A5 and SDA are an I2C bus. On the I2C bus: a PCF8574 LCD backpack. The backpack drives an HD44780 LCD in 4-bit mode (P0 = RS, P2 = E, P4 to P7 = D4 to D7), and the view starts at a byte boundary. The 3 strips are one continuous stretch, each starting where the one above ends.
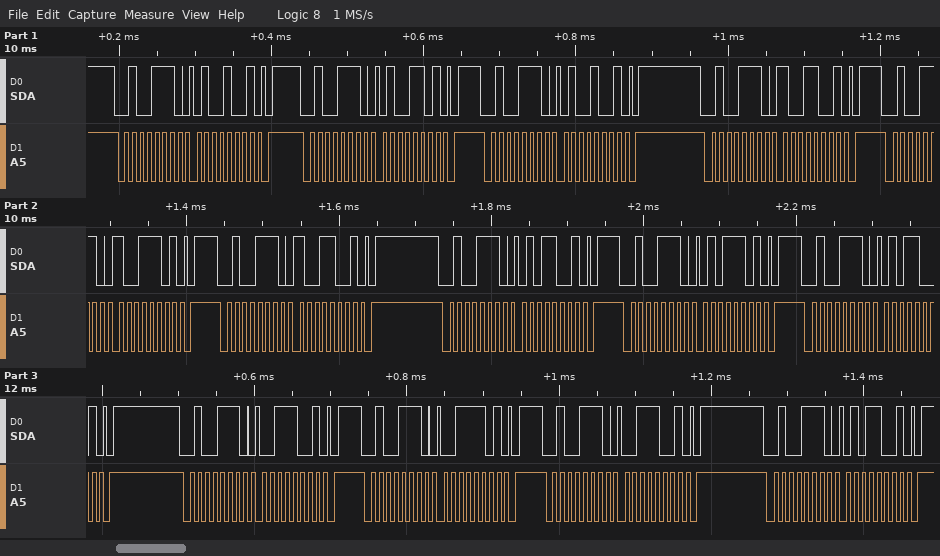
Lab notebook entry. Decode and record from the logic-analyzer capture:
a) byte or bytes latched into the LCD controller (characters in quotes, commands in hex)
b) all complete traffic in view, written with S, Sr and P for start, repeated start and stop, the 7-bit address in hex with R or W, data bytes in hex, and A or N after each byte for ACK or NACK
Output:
'I' 'S'
S 27W A 49 A P S 27W A 4D A P S 27W A 49 A P S 27W A 99 A P S 27W A 9D A P S 27W A 99 A P S 27W A 59 A P S 27W A 5D A P S 27W A 59 A P S 27W A 39 A P S 27W A 3D A P S 27W A 39 A P S 27W A 59 A P
